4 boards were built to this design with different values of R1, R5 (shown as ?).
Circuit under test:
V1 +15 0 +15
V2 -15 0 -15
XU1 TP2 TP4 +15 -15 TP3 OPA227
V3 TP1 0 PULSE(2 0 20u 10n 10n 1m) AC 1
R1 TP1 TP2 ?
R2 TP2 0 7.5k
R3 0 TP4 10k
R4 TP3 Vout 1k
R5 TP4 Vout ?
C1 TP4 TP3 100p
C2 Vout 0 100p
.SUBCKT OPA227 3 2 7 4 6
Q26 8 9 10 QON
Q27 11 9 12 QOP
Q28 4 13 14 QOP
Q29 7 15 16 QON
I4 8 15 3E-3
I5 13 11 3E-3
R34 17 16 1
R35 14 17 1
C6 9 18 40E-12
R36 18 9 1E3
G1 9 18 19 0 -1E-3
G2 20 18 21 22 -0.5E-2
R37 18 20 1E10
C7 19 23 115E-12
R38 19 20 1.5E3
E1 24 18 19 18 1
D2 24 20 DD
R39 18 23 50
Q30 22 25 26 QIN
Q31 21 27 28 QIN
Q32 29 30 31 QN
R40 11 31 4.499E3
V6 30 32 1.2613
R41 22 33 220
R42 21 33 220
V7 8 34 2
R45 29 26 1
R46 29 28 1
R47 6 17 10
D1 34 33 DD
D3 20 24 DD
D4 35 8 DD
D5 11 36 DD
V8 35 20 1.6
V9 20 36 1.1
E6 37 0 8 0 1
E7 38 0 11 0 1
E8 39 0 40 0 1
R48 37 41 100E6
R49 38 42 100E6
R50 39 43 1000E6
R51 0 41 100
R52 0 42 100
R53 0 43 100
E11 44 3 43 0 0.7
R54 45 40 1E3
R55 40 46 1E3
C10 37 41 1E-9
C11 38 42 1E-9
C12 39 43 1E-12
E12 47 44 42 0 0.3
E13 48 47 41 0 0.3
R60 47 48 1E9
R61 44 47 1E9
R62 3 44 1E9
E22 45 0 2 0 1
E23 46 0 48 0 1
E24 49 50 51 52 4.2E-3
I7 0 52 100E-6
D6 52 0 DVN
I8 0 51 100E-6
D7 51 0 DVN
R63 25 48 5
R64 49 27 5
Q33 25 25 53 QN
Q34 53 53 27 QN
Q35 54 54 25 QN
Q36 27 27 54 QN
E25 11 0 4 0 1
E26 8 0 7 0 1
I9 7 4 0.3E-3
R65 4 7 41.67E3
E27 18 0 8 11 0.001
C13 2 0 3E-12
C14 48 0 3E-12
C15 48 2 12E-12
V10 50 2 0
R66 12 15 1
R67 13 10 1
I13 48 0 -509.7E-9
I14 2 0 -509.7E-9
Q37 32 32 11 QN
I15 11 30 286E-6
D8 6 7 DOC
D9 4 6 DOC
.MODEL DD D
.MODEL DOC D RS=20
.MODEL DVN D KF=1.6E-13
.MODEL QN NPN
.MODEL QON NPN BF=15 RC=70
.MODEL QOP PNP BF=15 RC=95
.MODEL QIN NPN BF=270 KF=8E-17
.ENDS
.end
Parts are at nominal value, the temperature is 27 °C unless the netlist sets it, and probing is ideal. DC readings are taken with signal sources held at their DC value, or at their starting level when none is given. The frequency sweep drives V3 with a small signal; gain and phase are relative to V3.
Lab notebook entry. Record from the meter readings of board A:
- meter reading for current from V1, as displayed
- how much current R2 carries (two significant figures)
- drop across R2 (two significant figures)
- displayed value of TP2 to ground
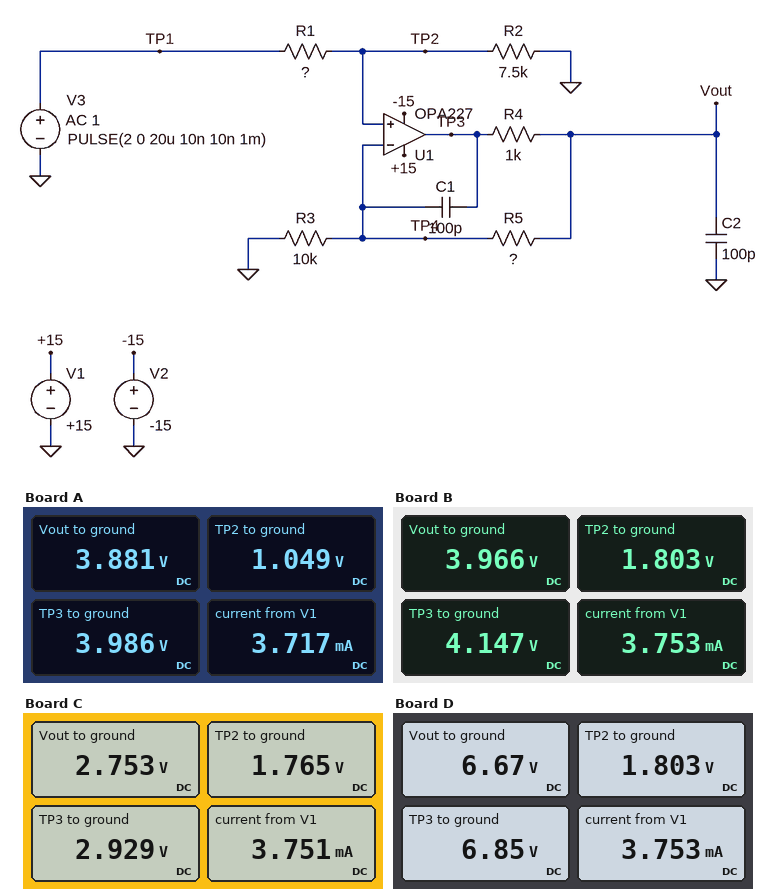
3.717 mA
140 µA
1.0 V
1.049 V
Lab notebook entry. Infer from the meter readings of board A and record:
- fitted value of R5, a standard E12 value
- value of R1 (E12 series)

27 kΩ
6.8 kΩ
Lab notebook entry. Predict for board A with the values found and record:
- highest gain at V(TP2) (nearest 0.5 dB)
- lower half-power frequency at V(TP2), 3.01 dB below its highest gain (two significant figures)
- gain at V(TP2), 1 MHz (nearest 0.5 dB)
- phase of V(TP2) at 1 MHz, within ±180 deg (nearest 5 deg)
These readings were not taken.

0 dB
2.6 MHz
-5.5 dB
-5 deg
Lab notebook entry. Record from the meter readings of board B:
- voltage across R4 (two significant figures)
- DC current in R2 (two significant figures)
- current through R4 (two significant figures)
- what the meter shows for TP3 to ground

180 mV
240 µA
180 µA
4.147 V
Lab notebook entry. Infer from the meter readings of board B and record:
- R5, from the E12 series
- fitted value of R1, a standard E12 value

12 kΩ
820 Ω
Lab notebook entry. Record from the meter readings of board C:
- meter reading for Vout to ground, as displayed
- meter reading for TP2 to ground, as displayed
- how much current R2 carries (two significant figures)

2.753 V
1.765 V
240 µA
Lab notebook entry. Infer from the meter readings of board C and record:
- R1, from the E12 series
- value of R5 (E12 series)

1 kΩ
5.6 kΩ
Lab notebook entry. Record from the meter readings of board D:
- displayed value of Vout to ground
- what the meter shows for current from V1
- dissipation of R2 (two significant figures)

6.67 V
3.753 mA
430 µW
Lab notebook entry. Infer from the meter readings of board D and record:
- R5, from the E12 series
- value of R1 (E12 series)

27 kΩ
820 Ω
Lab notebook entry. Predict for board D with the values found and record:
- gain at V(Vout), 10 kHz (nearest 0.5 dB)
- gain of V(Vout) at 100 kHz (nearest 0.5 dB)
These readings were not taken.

10.5 dB
5.5 dB
